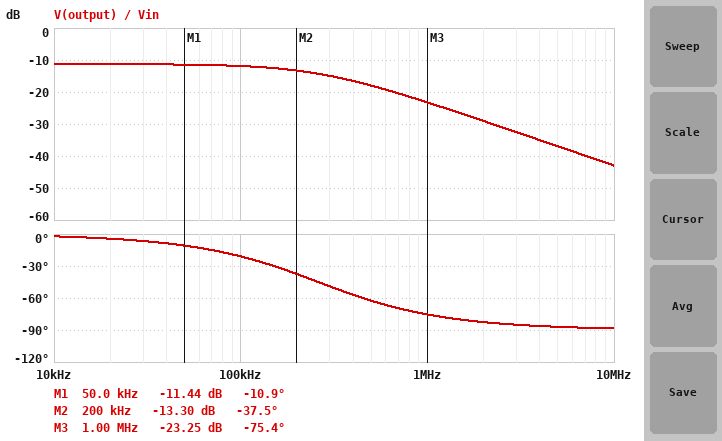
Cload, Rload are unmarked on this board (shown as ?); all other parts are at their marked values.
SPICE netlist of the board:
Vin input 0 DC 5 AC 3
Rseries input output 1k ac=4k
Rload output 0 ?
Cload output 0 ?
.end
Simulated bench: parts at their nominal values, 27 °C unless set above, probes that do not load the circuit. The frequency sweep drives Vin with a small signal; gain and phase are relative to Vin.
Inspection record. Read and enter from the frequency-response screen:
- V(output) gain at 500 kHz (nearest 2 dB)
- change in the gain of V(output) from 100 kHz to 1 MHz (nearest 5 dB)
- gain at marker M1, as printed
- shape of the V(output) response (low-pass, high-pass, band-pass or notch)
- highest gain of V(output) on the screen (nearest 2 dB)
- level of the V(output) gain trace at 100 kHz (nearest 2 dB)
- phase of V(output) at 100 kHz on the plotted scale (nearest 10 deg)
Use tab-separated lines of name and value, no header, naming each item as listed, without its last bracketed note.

V(output) gain at 500 kHz	-18 dB
change in the gain of V(output) from 100 kHz to 1 MHz	-10 dB
gain at marker M1, as printed	-11.44 dB
shape of the V(output) response	low-pass
highest gain of V(output) on the screen	-12 dB
level of the V(output) gain trace at 100 kHz	-12 dB
phase of V(output) at 100 kHz on the plotted scale	-20 deg
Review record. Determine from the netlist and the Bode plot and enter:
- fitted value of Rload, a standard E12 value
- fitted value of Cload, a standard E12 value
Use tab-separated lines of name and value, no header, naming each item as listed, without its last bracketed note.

fitted value of Rload, a standard E12 value	1.5 kΩ
fitted value of Cload, a standard E12 value	560 pF
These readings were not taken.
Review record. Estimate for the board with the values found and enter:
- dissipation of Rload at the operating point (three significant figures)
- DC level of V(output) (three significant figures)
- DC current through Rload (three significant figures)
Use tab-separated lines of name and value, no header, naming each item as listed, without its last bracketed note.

dissipation of Rload at the operating point	6.00 mW
DC level of V(output)	3.00 V
DC current through Rload	2.00 mA
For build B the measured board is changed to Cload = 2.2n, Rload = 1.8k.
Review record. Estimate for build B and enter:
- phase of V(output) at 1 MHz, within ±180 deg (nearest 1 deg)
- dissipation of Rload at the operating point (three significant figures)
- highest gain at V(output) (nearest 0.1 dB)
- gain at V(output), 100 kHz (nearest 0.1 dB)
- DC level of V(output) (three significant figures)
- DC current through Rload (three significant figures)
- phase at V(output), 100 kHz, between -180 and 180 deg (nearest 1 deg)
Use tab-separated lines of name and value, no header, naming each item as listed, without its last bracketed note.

phase of V(output) at 1 MHz, within ±180 deg	-87 deg
dissipation of Rload at the operating point	5.74 mW
highest gain at V(output)	-10.2 dB
gain at V(output), 100 kHz	-16.1 dB
DC level of V(output)	3.21 V
DC current through Rload	1.79 mA
phase at V(output), 100 kHz, between -180 and 180 deg	-60 deg
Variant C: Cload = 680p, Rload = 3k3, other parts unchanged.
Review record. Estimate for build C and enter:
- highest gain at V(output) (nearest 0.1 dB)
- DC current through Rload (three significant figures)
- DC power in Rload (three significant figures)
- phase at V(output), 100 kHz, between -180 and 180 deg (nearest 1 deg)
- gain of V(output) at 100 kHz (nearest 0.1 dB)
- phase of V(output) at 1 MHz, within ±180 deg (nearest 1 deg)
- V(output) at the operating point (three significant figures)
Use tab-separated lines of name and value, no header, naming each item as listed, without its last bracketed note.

highest gain at V(output)	-6.9 dB
DC current through Rload	1.16 mA
DC power in Rload	4.46 mW
phase at V(output), 100 kHz, between -180 and 180 deg	-38 deg
gain of V(output) at 100 kHz	-8.9 dB
phase of V(output) at 1 MHz, within ±180 deg	-83 deg
V(output) at the operating point	3.84 V
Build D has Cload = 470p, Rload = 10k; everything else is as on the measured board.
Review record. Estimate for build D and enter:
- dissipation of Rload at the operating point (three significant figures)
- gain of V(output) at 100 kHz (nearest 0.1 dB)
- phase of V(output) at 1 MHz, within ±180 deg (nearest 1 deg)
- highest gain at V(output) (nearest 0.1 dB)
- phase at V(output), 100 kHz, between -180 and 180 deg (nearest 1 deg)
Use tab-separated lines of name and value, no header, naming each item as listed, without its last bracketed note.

dissipation of Rload at the operating point	2.07 mW
gain of V(output) at 100 kHz	-5.3 dB
phase of V(output) at 1 MHz, within ±180 deg	-83 deg
highest gain at V(output)	-2.9 dB
phase at V(output), 100 kHz, between -180 and 180 deg	-40 deg
